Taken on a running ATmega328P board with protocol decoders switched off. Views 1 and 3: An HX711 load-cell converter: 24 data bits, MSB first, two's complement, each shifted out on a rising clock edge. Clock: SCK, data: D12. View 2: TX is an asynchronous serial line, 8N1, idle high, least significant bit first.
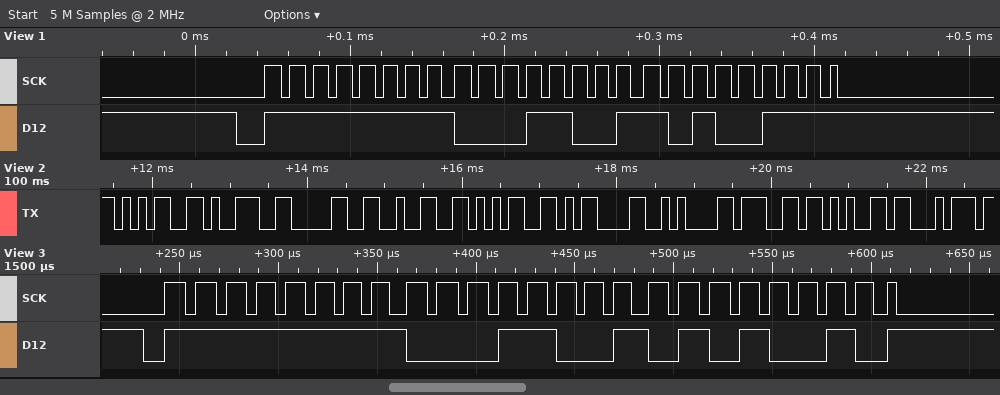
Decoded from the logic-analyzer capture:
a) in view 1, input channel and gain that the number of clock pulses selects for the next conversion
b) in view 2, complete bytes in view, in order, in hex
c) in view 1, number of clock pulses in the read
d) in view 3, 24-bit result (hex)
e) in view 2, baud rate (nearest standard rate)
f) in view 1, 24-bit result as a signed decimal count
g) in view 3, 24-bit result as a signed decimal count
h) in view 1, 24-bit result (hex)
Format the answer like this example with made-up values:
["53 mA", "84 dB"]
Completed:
["channel A, gain 128", "0x35 0x39 0x30 0x32 0x35 0x0D 0x0A 0x67 0x65 0x74", "25", "0xFF1952", "9600 baud", "-58969", "-59054", "0xFF19A7"]
